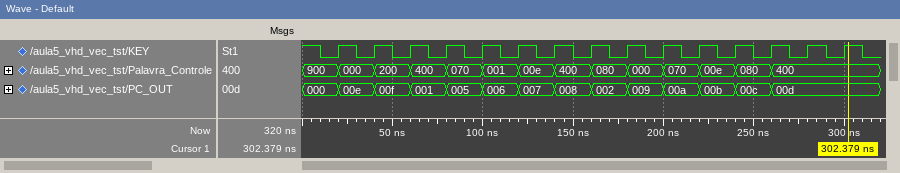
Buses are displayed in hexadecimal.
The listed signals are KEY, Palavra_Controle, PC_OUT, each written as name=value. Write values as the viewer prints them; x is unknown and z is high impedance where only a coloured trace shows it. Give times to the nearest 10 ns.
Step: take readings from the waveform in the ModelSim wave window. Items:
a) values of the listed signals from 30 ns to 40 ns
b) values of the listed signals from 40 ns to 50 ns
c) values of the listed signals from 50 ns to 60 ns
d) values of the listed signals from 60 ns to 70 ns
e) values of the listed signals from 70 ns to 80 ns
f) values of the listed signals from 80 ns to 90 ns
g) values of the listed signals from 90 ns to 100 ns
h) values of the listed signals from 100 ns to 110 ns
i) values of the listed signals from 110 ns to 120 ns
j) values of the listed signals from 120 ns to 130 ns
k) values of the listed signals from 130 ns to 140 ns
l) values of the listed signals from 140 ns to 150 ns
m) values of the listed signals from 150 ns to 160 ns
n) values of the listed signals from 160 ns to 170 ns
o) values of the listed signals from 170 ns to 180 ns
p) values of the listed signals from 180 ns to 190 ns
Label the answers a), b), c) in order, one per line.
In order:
a) KEY=0, Palavra_Controle=000, PC_OUT=00e
b) KEY=1, Palavra_Controle=200, PC_OUT=00f
c) KEY=0, Palavra_Controle=200, PC_OUT=00f
d) KEY=1, Palavra_Controle=400, PC_OUT=001
e) KEY=0, Palavra_Controle=400, PC_OUT=001
f) KEY=1, Palavra_Controle=070, PC_OUT=005
g) KEY=0, Palavra_Controle=070, PC_OUT=005
h) KEY=1, Palavra_Controle=001, PC_OUT=006
i) KEY=0, Palavra_Controle=001, PC_OUT=006
j) KEY=1, Palavra_Controle=00e, PC_OUT=007
k) KEY=0, Palavra_Controle=00e, PC_OUT=007
l) KEY=1, Palavra_Controle=400, PC_OUT=008
m) KEY=0, Palavra_Controle=400, PC_OUT=008
n) KEY=1, Palavra_Controle=080, PC_OUT=002
o) KEY=0, Palavra_Controle=080, PC_OUT=002
p) KEY=1, Palavra_Controle=000, PC_OUT=009
